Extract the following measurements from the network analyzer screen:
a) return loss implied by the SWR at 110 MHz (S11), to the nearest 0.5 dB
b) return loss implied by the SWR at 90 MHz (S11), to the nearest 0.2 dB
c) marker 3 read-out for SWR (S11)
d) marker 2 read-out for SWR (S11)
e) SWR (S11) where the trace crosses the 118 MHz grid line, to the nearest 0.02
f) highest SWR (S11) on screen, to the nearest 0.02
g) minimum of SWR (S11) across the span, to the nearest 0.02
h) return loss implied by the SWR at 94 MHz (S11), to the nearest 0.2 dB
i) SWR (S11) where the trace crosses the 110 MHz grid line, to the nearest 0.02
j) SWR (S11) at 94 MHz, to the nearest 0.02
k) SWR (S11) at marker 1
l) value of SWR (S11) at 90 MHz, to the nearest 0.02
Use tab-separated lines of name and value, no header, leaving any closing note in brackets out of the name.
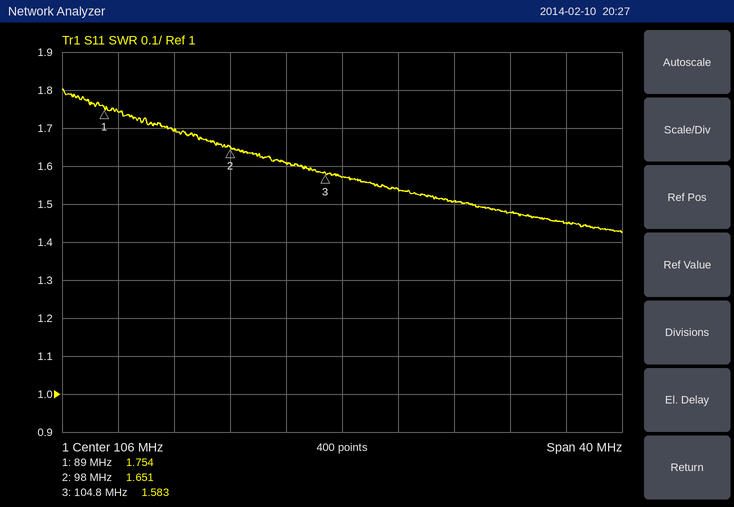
return loss implied by the SWR at 110 MHz (S11), to the nearest 0.5 dB	13.5 dB
return loss implied by the SWR at 90 MHz (S11), to the nearest 0.2 dB	11.4 dB
marker 3 read-out for SWR	1.583
marker 2 read-out for SWR	1.651
SWR (S11) where the trace crosses the 118 MHz grid line, to the nearest 0.02	1.48
highest SWR (S11) on screen, to the nearest 0.02	1.80
minimum of SWR (S11) across the span, to the nearest 0.02	1.42
return loss implied by the SWR at 94 MHz (S11), to the nearest 0.2 dB	11.8 dB
SWR (S11) where the trace crosses the 110 MHz grid line, to the nearest 0.02	1.54
SWR (S11) at 94 MHz, to the nearest 0.02	1.70
SWR (S11) at marker 1	1.754
value of SWR (S11) at 90 MHz, to the nearest 0.02	1.74
